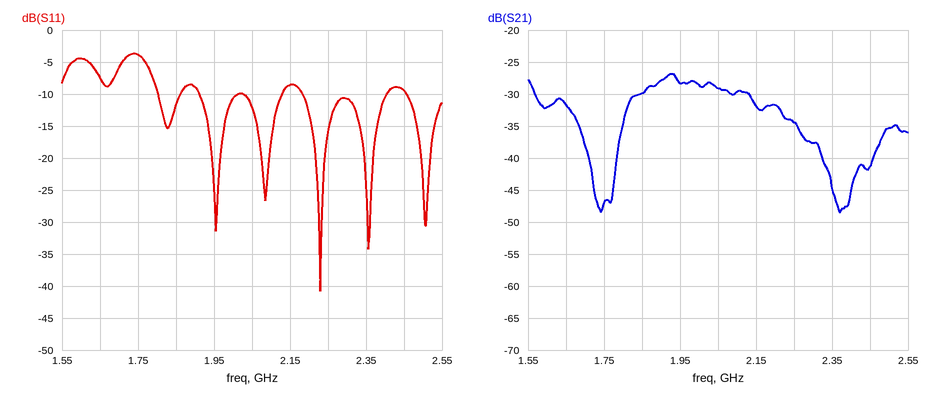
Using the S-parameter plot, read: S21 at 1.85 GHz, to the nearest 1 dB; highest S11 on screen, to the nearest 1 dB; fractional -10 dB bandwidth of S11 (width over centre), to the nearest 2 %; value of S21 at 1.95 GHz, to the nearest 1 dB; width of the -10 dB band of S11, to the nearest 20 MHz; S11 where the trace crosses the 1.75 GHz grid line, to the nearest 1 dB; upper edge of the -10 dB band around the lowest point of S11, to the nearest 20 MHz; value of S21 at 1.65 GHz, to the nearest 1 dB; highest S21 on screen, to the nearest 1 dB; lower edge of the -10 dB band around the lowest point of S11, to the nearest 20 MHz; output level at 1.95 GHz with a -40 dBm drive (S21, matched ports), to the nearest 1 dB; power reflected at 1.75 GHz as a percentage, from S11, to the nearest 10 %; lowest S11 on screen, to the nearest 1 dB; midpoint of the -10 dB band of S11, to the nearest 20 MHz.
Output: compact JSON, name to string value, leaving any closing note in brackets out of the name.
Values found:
{"S21 at 1.85 GHz, to the nearest 1 dB": "-30 dB", "highest S11 on screen, to the nearest 1 dB": "-4 dB", "fractional -10 dB bandwidth of S11 (width over centre), to the nearest 2 %": "10 %", "value of S21 at 1.95 GHz, to the nearest 1 dB": "-28 dB", "width of the -10 dB band of S11, to the nearest 20 MHz": "220 MHz", "S11 where the trace crosses the 1.75 GHz grid line, to the nearest 1 dB": "-4 dB", "upper edge of the -10 dB band around the lowest point of S11, to the nearest 20 MHz": "2.40 GHz", "value of S21 at 1.65 GHz, to the nearest 1 dB": "-32 dB", "highest S21 on screen, to the nearest 1 dB": "-27 dB", "lower edge of the -10 dB band around the lowest point of S11, to the nearest 20 MHz": "2.18 GHz", "output level at 1.95 GHz with a -40 dBm drive (S21, matched ports), to the nearest 1 dB": "-68 dBm", "power reflected at 1.75 GHz as a percentage, from S11, to the nearest 10 %": "40 %", "lowest S11 on screen, to the nearest 1 dB": "-41 dB", "midpoint of the -10 dB band of S11, to the nearest 20 MHz": "2.30 GHz"}
